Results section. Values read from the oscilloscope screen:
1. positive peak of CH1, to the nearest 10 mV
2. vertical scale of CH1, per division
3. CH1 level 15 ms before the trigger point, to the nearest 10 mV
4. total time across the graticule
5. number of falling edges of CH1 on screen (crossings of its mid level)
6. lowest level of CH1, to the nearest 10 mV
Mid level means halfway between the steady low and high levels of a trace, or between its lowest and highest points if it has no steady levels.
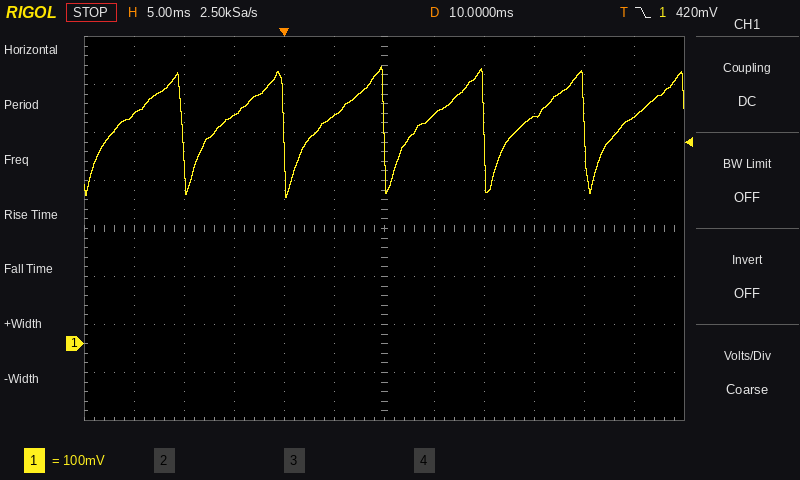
580 mV
100 mV
480 mV
60 ms
5
300 mV
